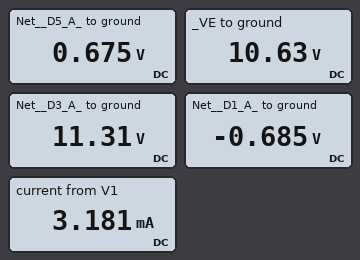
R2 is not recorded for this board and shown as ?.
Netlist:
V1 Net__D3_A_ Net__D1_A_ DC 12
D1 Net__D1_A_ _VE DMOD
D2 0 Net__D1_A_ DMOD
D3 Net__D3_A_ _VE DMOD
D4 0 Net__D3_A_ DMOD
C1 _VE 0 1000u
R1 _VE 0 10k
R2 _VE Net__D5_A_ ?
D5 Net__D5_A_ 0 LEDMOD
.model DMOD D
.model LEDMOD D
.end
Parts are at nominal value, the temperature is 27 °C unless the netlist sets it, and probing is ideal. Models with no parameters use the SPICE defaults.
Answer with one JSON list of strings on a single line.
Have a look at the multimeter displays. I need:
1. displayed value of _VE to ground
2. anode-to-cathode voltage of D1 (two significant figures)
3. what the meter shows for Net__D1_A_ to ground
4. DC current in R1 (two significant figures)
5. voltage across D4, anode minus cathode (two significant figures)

["10.63 V", "-11 V", "-0.685 V", "1.1 mA", "-11 V"]
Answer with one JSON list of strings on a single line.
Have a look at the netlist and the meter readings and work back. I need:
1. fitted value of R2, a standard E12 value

["4.7 kΩ"]
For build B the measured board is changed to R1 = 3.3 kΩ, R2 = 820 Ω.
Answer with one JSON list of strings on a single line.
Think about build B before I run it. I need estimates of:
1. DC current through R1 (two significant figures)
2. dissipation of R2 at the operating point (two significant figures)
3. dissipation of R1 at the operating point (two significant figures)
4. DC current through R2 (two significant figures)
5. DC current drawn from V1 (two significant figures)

["3.2 mA", "120 mW", "34 mW", "12 mA", "15 mA"]
